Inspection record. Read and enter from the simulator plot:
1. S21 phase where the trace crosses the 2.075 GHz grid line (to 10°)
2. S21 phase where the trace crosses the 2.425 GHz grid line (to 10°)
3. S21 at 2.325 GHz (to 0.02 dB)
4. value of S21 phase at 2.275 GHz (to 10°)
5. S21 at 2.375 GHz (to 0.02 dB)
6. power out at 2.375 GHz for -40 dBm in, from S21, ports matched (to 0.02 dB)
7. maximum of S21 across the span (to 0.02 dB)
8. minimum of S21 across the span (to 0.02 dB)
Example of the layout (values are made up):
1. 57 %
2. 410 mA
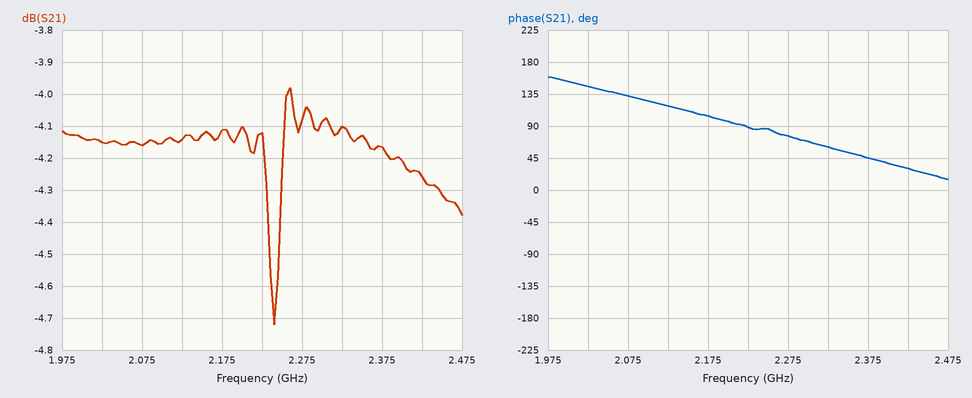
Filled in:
1. 130°
2. 30°
3. -4.10 dB
4. 80°
5. -4.16 dB
6. -44.16 dBm
7. -3.98 dB
8. -4.72 dB
